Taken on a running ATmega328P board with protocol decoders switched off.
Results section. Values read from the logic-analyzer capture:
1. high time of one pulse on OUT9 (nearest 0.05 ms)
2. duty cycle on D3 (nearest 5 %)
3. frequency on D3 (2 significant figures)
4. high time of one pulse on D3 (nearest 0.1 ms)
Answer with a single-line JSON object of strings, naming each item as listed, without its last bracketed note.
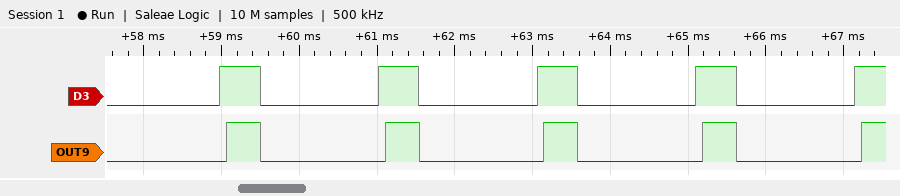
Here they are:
{"high time of one pulse on OUT9": "0.45 ms", "duty cycle on D3": "25 %", "frequency on D3": "490 Hz", "high time of one pulse on D3": "0.5 ms"}
